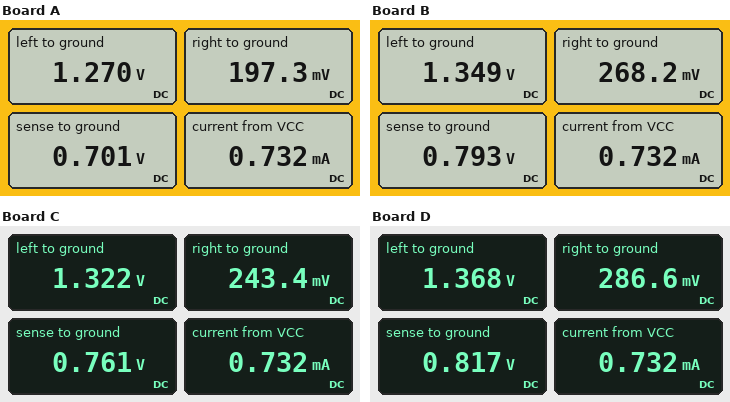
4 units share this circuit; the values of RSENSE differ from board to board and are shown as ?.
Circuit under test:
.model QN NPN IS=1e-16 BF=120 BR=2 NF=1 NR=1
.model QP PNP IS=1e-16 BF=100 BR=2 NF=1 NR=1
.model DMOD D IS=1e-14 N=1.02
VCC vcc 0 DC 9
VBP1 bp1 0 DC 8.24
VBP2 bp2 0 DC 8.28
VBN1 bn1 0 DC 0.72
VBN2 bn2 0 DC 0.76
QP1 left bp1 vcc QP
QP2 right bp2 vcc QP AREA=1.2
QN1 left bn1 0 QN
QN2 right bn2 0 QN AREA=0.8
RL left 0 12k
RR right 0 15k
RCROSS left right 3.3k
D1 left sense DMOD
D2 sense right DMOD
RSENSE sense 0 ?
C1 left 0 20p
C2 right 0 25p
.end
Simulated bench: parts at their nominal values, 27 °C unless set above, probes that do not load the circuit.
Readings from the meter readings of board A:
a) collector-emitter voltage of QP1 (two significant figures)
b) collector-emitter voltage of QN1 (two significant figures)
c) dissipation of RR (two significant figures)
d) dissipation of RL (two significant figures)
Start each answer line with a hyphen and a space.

- -7.7 V
- 1.3 V
- 2.6 µW
- 130 µW
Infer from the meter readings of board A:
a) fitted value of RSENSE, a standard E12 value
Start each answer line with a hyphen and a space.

- 33 kΩ
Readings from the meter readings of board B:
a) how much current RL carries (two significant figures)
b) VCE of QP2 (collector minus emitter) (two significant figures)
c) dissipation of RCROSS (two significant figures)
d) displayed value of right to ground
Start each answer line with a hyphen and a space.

- 110 µA
- -8.7 V
- 350 µW
- 268.2 mV
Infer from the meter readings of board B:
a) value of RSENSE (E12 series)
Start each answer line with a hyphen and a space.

- 82 kΩ
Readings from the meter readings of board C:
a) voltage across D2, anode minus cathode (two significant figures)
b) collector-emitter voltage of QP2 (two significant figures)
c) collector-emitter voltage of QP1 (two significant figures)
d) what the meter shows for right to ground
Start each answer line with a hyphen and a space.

- 520 mV
- -8.8 V
- -7.7 V
- 243.4 mV
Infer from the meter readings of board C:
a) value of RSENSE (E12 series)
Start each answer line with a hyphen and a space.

- 56 kΩ
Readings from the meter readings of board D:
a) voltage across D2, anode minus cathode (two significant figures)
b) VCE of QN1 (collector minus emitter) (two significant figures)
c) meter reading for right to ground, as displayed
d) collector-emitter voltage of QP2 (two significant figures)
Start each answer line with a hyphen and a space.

- 530 mV
- 1.4 V
- 286.6 mV
- -8.7 V
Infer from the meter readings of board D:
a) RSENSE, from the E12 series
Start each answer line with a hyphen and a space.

- 120 kΩ
